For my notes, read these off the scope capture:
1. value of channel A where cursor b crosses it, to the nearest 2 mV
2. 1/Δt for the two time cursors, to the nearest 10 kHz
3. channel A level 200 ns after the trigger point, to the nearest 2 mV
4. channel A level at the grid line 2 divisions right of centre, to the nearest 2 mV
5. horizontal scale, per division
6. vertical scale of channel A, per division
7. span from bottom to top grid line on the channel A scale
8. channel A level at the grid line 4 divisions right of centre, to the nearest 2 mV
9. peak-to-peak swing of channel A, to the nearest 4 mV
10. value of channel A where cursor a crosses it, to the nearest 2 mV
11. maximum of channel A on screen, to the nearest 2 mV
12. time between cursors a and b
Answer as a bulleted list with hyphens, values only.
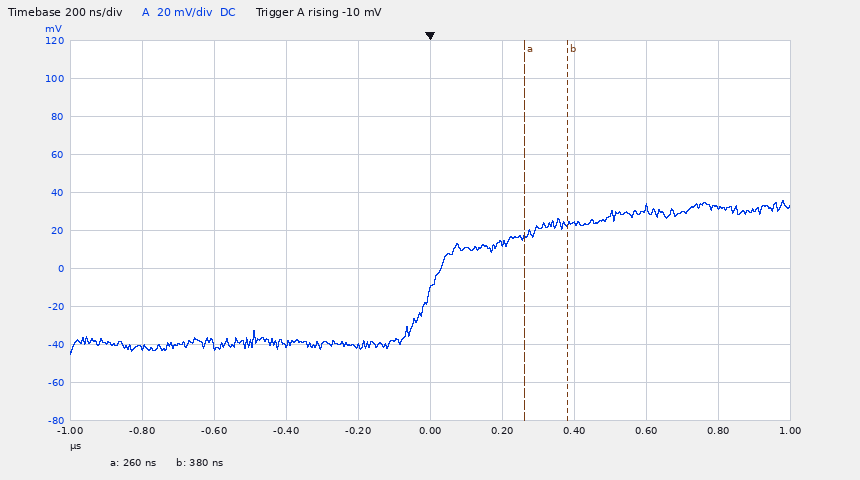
- 24 mV
- 8.33 MHz
- 14 mV
- 24 mV
- 200 ns
- 20 mV
- 200 mV
- 32 mV
- 80 mV
- 16 mV
- 36 mV
- 120 ns
